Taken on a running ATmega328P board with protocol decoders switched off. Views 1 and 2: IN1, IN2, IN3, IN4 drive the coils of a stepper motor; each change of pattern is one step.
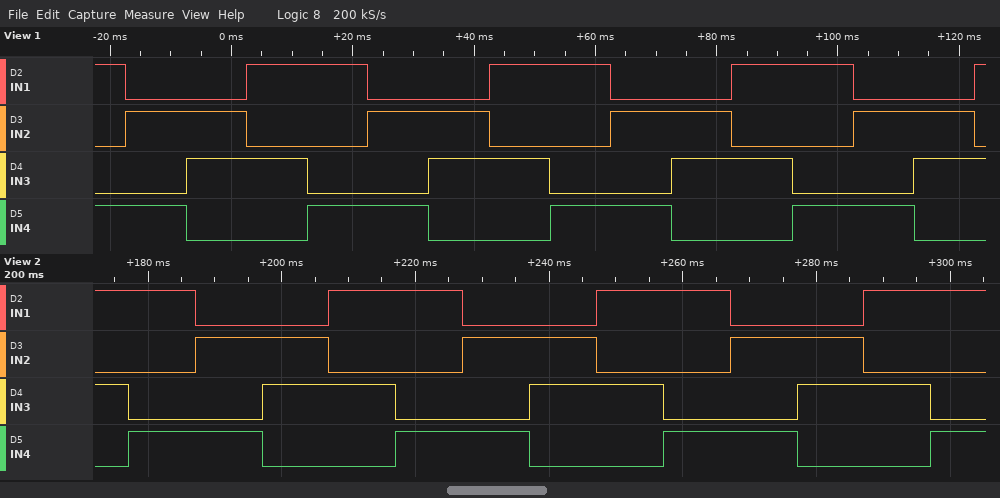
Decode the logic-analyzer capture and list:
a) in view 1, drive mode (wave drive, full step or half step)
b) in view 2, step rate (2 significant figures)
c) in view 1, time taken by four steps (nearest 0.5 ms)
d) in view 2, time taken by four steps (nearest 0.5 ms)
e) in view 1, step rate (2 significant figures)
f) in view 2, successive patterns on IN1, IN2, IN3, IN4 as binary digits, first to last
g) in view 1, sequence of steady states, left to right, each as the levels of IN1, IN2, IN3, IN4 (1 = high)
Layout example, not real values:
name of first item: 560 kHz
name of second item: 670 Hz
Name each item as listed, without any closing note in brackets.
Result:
in view 1, drive mode: full step
in view 2, step rate: 100 steps/s
in view 1, time taken by four steps: 40.0 ms
in view 2, time taken by four steps: 40.0 ms
in view 1, step rate: 100 steps/s
in view 2, successive patterns on IN1, IN2, IN3, IN4 as binary digits, first to last: 1010 1001 0101 0110 1010 1001 0101 0110 1010 1001 0101 0110 1010 1001
in view 1, sequence of steady states, left to right, each as the levels of IN1, IN2, IN3, IN4: 1001 0101 0110 1010 1001 0101 0110 1010 1001 0101 0110 1010 1001 0101 0110 1010
